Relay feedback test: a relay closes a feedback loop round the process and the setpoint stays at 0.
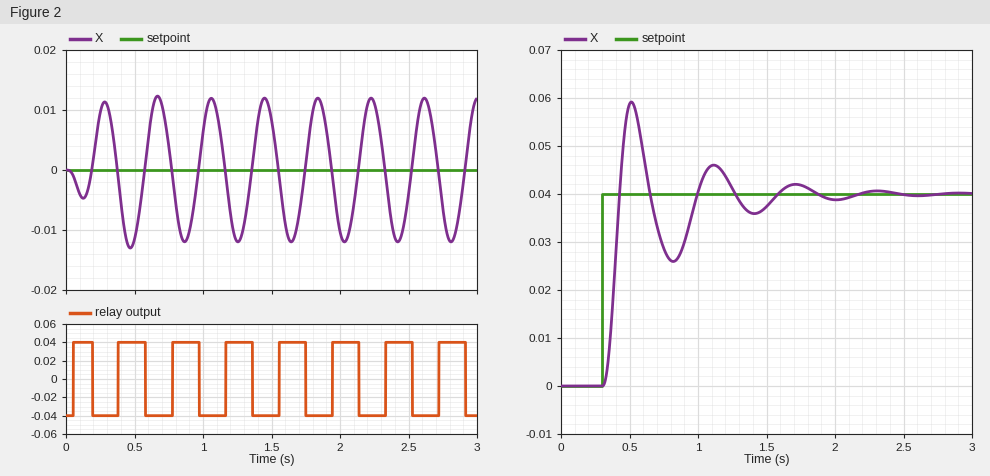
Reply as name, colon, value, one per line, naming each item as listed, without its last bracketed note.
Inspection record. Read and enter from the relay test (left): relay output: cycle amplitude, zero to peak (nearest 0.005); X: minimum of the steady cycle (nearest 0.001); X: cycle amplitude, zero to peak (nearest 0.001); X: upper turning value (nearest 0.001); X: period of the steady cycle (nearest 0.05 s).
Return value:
relay output: cycle amplitude, zero to peak: 0.040
X: minimum of the steady cycle: -0.012
X: cycle amplitude, zero to peak: 0.012
X: upper turning value: 0.012
X: period of the steady cycle: 0.40 s
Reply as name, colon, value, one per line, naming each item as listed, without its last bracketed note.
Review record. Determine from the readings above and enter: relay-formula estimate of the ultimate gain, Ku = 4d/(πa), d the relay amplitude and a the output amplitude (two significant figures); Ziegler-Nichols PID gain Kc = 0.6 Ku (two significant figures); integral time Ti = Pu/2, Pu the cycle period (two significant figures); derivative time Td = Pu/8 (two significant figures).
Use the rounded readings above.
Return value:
relay-formula estimate of the ultimate gain, Ku = 4d/(πa), d the relay amplitude and a the output amplitude: 4.2
Ziegler-Nichols PID gain Kc = 0.6 Ku: 2.5
integral time Ti = Pu/2, Pu the cycle period: 0.20 s
derivative time Td = Pu/8: 0.050 s
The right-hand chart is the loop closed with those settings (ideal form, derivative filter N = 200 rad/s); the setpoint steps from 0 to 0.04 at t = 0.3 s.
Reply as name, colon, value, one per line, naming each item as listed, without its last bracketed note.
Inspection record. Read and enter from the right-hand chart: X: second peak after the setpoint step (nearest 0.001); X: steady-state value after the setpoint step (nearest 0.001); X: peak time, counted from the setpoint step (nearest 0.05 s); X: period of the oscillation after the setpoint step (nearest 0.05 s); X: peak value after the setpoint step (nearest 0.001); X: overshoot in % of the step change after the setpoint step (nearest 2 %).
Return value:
X: second peak after the setpoint step: 0.046
X: steady-state value after the setpoint step: 0.040
X: peak time, counted from the setpoint step: 0.20 s
X: period of the oscillation after the setpoint step: 0.60 s
X: peak value after the setpoint step: 0.059
X: overshoot in % of the step change after the setpoint step: 48 %
